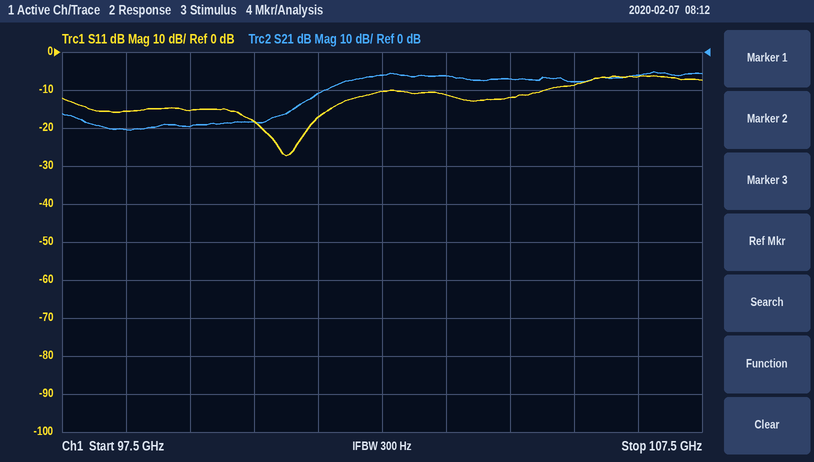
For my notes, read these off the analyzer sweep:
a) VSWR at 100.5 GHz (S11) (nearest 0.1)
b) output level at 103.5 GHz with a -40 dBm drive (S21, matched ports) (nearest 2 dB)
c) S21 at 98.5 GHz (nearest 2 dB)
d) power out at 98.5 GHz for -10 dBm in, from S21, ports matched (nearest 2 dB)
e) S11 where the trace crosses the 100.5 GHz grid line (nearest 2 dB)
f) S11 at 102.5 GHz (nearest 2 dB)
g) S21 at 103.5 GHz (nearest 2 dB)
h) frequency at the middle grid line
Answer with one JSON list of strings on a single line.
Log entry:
["1.3", "-46 dBm", "-20 dB", "-30 dBm", "-18 dB", "-10 dB", "-6 dB", "102.5 GHz"]
